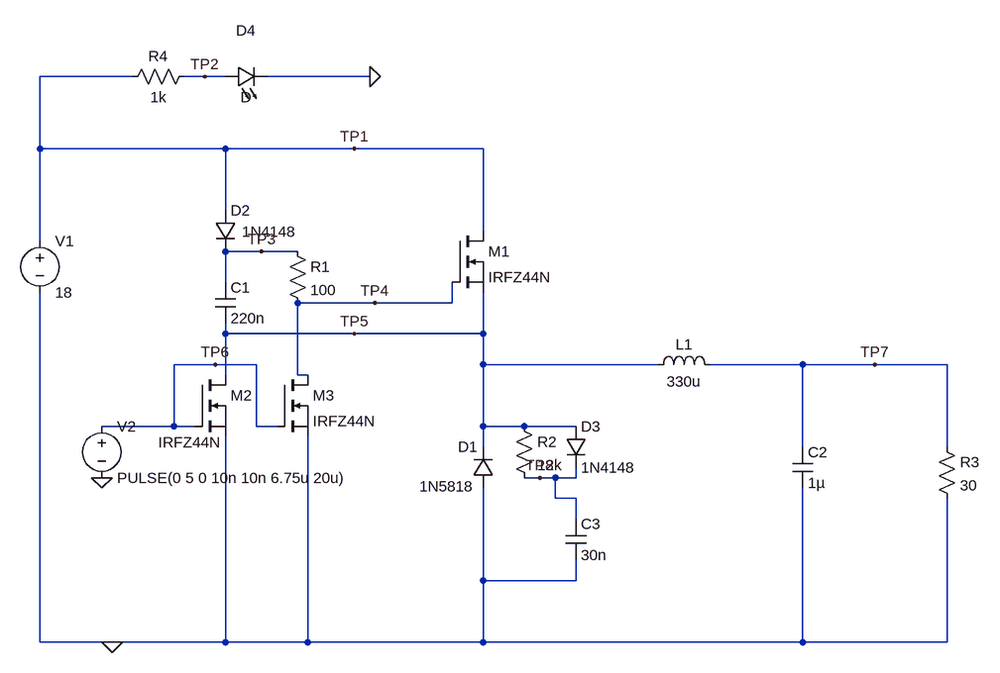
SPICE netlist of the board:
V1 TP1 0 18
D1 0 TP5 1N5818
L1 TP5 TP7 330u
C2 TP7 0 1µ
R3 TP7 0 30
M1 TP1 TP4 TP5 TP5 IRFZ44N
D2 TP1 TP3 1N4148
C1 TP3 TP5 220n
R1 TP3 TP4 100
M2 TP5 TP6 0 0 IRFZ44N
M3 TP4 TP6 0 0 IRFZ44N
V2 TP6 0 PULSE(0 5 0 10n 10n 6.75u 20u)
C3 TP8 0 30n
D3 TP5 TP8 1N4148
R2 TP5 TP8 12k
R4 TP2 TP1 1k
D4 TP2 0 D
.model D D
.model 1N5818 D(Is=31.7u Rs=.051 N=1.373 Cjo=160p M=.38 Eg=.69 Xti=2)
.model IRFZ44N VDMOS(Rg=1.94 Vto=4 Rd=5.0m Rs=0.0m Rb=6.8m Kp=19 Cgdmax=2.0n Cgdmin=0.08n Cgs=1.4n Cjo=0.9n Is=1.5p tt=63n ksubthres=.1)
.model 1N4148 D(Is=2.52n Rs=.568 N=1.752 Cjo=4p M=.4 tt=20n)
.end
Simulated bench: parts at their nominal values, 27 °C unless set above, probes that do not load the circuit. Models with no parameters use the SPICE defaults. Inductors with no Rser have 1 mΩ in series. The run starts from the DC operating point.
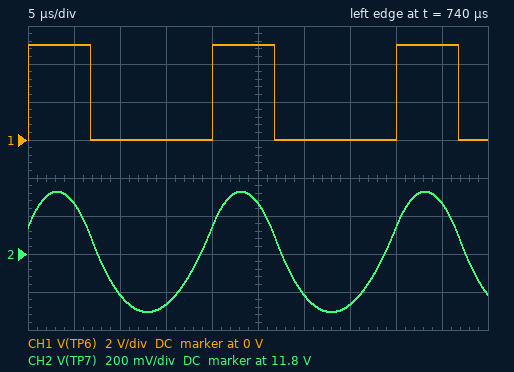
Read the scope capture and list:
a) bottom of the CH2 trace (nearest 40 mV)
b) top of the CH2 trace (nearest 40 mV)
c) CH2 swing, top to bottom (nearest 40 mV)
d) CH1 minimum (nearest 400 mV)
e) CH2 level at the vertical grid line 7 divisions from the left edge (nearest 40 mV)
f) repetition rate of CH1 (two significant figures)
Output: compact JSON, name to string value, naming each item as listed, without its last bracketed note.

{"bottom of the CH2 trace": "11.48 V", "top of the CH2 trace": "12.12 V", "CH2 swing, top to bottom": "640 mV", "CH1 minimum": "0 V", "CH2 level at the vertical grid line 7 divisions from the left edge": "11.52 V", "repetition rate of CH1": "50 kHz"}
